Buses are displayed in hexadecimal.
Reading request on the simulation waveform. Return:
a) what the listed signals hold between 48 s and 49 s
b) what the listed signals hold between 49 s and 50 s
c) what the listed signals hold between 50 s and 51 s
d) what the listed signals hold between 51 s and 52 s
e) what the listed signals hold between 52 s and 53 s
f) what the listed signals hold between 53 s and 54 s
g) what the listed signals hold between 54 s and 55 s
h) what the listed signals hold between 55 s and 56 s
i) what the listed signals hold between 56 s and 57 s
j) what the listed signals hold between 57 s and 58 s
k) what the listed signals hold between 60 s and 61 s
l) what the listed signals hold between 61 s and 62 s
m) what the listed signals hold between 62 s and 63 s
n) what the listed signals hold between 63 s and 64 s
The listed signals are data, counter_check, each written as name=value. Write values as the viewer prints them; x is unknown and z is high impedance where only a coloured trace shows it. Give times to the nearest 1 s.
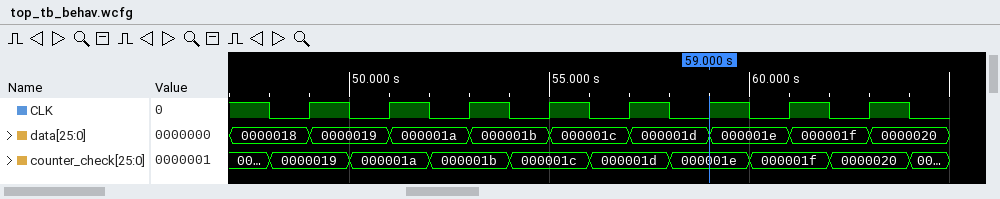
data=0000018, counter_check=0000019
data=0000019, counter_check=0000019
data=0000019, counter_check=000001a
data=000001a, counter_check=000001a
data=000001a, counter_check=000001b
data=000001b, counter_check=000001b
data=000001b, counter_check=000001c
data=000001c, counter_check=000001c
data=000001c, counter_check=000001d
data=000001d, counter_check=000001d
data=000001e, counter_check=000001f
data=000001f, counter_check=000001f
data=000001f, counter_check=0000020
data=0000020, counter_check=0000020
